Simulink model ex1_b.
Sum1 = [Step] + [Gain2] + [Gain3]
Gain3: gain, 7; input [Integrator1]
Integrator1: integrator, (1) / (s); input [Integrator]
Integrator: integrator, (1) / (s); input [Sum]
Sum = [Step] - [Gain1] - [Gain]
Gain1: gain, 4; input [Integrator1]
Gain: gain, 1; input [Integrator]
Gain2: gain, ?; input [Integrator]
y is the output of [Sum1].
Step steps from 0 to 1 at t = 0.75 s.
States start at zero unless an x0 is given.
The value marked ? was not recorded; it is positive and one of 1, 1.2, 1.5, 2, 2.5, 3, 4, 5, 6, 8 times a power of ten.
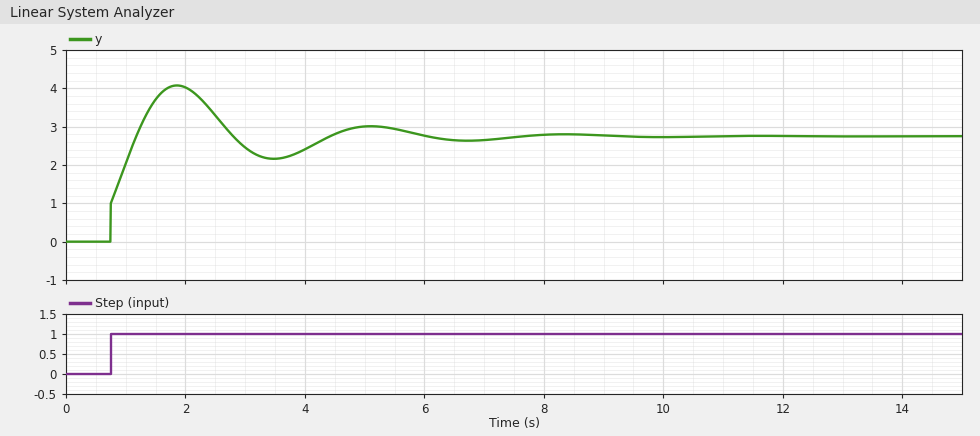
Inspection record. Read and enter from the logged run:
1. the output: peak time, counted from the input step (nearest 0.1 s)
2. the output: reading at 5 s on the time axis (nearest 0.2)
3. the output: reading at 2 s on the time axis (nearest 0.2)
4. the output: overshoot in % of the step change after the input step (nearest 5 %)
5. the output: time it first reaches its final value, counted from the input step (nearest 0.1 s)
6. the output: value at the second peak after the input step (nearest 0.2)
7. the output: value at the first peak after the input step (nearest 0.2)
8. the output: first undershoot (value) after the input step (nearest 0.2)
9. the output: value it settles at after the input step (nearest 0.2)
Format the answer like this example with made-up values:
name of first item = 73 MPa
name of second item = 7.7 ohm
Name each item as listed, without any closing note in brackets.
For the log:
the output: peak time, counted from the input step = 1.1 s
the output: reading at 5 s on the time axis = 3.0
the output: reading at 2 s on the time axis = 4.0
the output: overshoot in % of the step change after the input step = 50 %
the output: time it first reaches its final value, counted from the input step = 0.4 s
the output: value at the second peak after the input step = 3.0
the output: value at the first peak after the input step = 4.0
the output: first undershoot (value) after the input step = 2.2
the output: value it settles at after the input step = 2.8
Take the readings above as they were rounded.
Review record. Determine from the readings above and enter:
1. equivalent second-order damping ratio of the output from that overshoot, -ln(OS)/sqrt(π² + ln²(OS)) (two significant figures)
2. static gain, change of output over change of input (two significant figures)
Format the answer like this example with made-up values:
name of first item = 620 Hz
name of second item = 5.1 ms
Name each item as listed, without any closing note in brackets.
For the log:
equivalent second-order damping ratio of the output from that overshoot, -ln(OS)/sqrt(π² + ln²(OS)) = 0.22
static gain, change of output over change of input = 2.8
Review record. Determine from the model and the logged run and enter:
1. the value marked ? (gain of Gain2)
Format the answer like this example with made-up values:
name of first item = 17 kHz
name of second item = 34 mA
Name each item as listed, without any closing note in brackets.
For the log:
the value marked ? = 4
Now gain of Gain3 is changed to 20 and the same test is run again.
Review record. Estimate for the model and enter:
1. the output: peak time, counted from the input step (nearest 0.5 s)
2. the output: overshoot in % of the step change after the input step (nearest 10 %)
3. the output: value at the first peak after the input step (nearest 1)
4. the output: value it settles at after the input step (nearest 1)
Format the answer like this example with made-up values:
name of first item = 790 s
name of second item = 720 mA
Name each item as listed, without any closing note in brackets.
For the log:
the output: peak time, counted from the input step = 1.5 s
the output: overshoot in % of the step change after the input step = 40 %
the output: value at the first peak after the input step = 8
the output: value it settles at after the input step = 6
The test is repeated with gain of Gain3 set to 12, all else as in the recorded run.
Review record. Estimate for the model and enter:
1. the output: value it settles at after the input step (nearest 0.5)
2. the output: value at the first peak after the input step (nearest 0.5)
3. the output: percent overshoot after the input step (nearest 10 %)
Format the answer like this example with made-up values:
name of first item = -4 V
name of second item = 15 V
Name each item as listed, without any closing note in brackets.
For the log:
the output: value it settles at after the input step = 4.0
the output: value at the first peak after the input step = 5.5
the output: percent overshoot after the input step = 40 %
